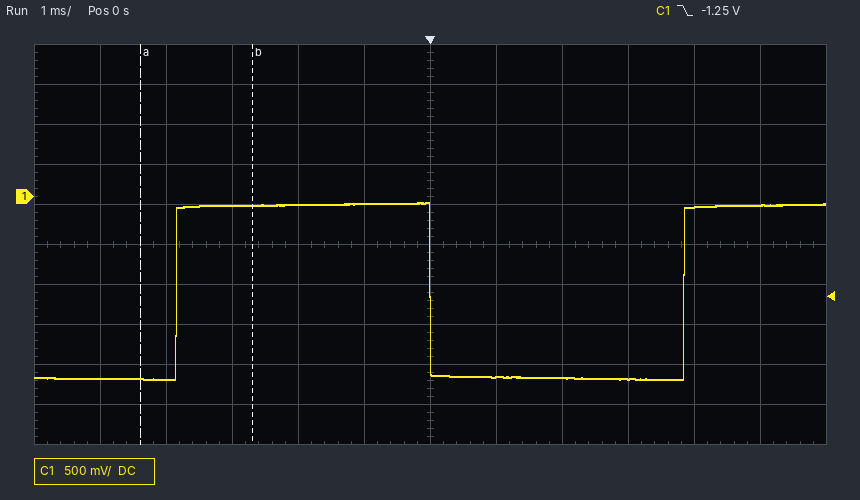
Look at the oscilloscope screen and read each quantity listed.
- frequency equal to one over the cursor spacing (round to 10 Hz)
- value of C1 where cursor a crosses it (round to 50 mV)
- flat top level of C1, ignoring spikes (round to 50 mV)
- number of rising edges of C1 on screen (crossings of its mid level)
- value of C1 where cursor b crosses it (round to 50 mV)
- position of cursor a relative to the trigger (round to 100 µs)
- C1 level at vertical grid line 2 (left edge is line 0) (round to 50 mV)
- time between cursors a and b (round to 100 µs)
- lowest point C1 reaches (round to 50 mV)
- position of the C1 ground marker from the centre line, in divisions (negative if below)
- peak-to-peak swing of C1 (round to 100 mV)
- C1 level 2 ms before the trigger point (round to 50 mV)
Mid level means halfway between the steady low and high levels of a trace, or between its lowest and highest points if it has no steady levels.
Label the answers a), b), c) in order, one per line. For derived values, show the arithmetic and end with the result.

a) 1 / 1.7 ms ≈ 590 Hz
b) -2.30 V
c) -100 mV
d) 2
e) -100 mV
f) -4.4 ms
g) -2.30 V
h) 1.7 ms
i) -2.30 V
j) +1.2 div
k) 2.20 V
l) -100 mV
